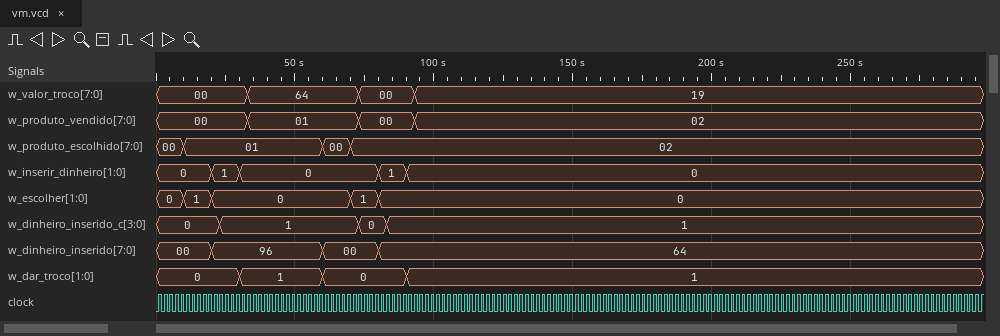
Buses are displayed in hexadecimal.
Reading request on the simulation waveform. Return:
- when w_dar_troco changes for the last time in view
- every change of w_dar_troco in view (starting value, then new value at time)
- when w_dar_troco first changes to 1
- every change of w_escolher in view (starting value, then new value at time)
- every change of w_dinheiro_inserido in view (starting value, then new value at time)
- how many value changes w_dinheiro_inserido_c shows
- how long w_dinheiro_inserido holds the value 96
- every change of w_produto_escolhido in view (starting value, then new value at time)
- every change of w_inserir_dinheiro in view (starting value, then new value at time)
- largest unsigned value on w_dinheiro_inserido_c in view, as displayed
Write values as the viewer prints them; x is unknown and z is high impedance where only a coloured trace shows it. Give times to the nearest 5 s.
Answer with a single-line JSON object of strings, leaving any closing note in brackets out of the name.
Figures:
{"when w_dar_troco changes for the last time in view": "90 s", "every change of w_dar_troco in view": "0, 1 at 30 s, 0 at 60 s, 1 at 90 s", "when w_dar_troco first changes to 1": "30 s", "every change of w_escolher in view": "0, 1 at 10 s, 0 at 20 s, 1 at 70 s, 0 at 80 s", "every change of w_dinheiro_inserido in view": "00, 96 at 20 s, 00 at 60 s, 64 at 80 s", "how many value changes w_dinheiro_inserido_c shows": "3", "how long w_dinheiro_inserido holds the value 96": "40 s", "every change of w_produto_escolhido in view": "00, 01 at 10 s, 00 at 60 s, 02 at 70 s", "every change of w_inserir_dinheiro in view": "0, 1 at 20 s, 0 at 30 s, 1 at 80 s, 0 at 90 s", "largest unsigned value on w_dinheiro_inserido_c in view, as displayed": "1"}
